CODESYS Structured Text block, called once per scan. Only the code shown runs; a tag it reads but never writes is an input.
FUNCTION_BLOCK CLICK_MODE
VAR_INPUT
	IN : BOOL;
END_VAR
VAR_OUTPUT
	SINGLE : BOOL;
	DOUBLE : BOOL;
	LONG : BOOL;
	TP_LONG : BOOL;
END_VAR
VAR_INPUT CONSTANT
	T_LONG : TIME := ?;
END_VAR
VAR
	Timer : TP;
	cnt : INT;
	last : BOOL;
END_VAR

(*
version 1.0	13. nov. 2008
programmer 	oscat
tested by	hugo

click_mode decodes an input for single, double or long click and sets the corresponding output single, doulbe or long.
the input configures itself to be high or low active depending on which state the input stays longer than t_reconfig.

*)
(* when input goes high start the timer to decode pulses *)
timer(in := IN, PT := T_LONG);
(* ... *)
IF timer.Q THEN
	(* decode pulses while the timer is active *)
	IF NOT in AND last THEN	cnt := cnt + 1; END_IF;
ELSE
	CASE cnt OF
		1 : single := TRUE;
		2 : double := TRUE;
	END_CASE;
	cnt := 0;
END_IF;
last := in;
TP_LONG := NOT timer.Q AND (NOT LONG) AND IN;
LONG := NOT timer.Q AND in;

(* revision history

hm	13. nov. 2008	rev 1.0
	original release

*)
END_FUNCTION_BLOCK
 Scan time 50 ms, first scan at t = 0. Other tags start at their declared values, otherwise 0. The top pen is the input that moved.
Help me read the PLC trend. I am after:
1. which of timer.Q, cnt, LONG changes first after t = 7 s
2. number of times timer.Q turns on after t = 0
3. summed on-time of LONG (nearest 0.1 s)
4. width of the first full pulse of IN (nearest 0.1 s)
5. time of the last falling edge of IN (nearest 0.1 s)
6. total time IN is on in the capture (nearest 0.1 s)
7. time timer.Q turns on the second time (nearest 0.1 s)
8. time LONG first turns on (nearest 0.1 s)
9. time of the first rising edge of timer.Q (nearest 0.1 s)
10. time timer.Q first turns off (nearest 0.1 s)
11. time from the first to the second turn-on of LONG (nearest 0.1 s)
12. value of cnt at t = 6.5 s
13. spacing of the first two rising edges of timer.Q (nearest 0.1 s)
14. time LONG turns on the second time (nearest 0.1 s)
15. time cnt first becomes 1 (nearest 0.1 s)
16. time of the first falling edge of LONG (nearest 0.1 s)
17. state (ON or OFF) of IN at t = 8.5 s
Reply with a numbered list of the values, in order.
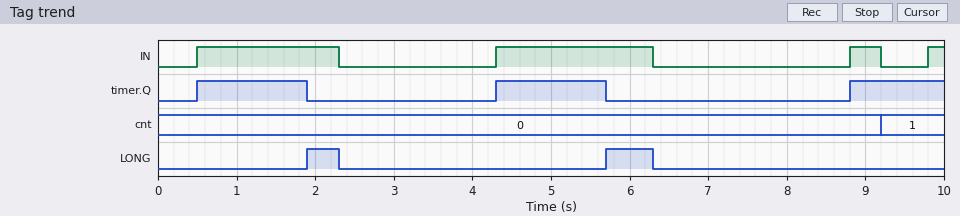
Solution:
1. timer.Q
2. 3
3. 1.0 s
4. 1.8 s
5. 9.2 s
6. 4.4 s
7. 4.3 s
8. 1.9 s
9. 0.5 s
10. 1.9 s
11. 3.8 s
12. 0
13. 3.8 s
14. 5.7 s
15. 9.2 s
16. 2.3 s
17. OFF
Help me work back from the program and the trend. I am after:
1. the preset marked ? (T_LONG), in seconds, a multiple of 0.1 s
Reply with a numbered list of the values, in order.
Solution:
1. 1.4 s
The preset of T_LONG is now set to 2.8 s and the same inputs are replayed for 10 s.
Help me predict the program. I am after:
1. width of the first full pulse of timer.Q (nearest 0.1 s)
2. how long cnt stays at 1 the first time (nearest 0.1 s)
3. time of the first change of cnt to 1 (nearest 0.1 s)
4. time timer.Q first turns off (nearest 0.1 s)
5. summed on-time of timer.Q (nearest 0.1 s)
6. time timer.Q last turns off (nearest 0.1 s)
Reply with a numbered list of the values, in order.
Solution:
1. 2.8 s
2. 1.0 s
3. 2.3 s
4. 3.3 s
5. 6.8 s
6. 7.1 s
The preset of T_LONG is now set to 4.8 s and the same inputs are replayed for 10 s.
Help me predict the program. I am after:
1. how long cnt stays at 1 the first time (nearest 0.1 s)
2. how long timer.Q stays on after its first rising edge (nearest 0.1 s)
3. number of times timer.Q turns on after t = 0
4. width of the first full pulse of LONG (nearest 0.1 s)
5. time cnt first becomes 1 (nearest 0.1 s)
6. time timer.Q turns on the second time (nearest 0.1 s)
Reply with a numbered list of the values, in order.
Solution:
1. 3.0 s
2. 4.8 s
3. 2
4. 1.0 s
5. 2.3 s
6. 8.8 s
